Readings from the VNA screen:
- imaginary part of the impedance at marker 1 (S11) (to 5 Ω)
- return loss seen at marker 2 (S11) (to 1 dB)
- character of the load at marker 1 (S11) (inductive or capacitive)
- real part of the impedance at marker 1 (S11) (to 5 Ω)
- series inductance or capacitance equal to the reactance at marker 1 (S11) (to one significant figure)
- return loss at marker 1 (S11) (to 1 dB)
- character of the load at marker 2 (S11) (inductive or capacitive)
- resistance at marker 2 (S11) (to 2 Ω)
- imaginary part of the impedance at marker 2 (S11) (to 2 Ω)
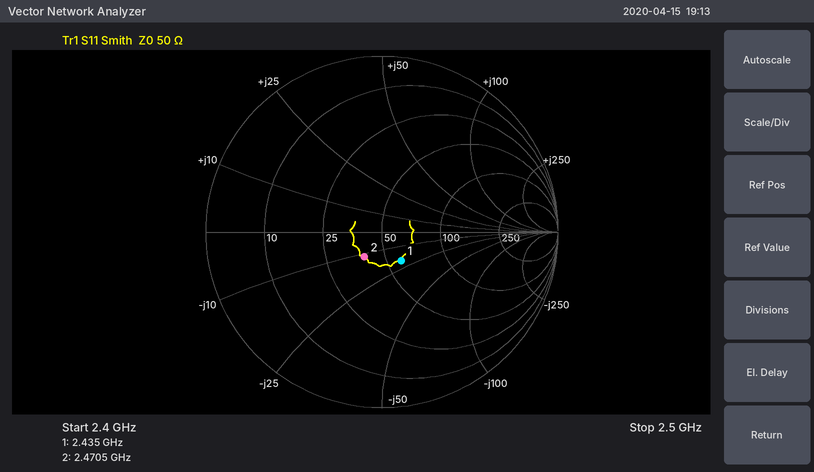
-20 Ω
15 dB
capacitive
60 Ω
3 pF
14 dB
capacitive
40 Ω
-12 Ω
